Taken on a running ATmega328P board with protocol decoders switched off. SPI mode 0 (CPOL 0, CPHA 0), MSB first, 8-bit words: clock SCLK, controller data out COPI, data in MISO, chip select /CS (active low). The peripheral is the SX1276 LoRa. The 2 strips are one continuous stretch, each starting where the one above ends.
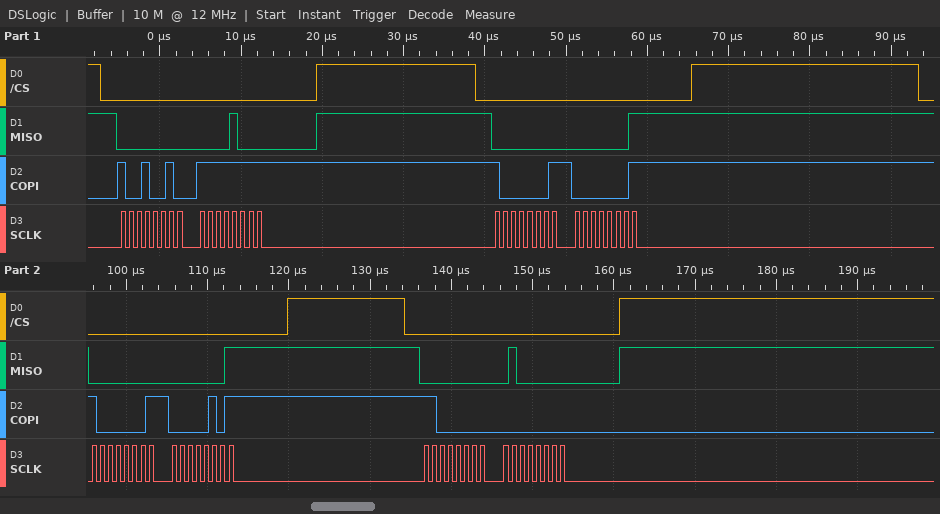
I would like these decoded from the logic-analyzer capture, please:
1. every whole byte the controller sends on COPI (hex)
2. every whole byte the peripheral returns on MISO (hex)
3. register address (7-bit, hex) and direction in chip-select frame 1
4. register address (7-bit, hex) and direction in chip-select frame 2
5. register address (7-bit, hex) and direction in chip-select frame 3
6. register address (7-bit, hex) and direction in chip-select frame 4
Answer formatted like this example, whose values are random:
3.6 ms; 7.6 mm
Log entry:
0x92 0xFF 0x81 0x01 0x81 0x05 0xC0 0x00; 0x00 0x08 0x00 0x01 0x00 0x01 0x00 0x40; 0x12 write; 0x01 write; 0x01 write; 0x40 write
